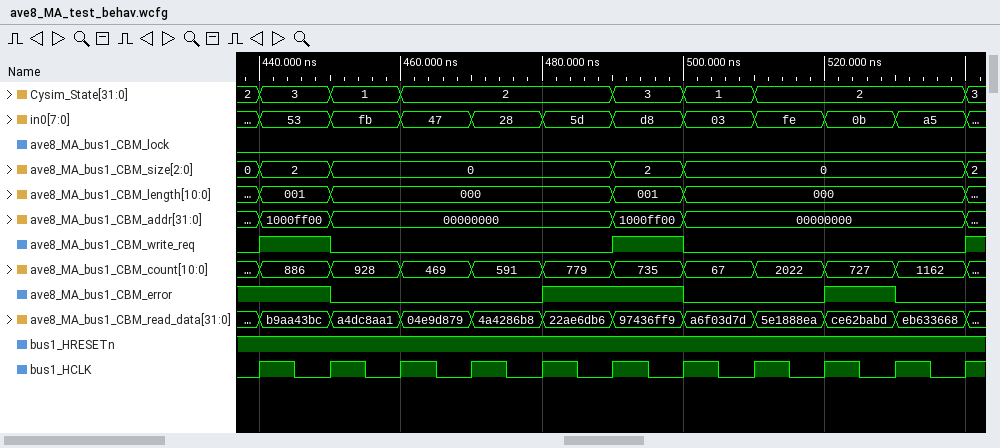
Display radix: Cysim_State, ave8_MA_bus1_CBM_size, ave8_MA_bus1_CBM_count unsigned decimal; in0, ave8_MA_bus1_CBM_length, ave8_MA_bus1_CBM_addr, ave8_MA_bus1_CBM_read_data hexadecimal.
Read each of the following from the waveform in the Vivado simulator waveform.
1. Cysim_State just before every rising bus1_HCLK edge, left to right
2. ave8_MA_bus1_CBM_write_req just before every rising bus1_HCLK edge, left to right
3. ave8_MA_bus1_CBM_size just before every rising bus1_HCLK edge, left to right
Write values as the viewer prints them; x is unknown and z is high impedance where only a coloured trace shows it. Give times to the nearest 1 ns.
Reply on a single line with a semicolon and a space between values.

2, 3, 1, 2, 2, 2, 3, 1, 2, 2, 2; 0 1 0 0 0 0 1 0 0 0 0; 0, 2, 0, 0, 0, 0, 2, 0, 0, 0, 0
